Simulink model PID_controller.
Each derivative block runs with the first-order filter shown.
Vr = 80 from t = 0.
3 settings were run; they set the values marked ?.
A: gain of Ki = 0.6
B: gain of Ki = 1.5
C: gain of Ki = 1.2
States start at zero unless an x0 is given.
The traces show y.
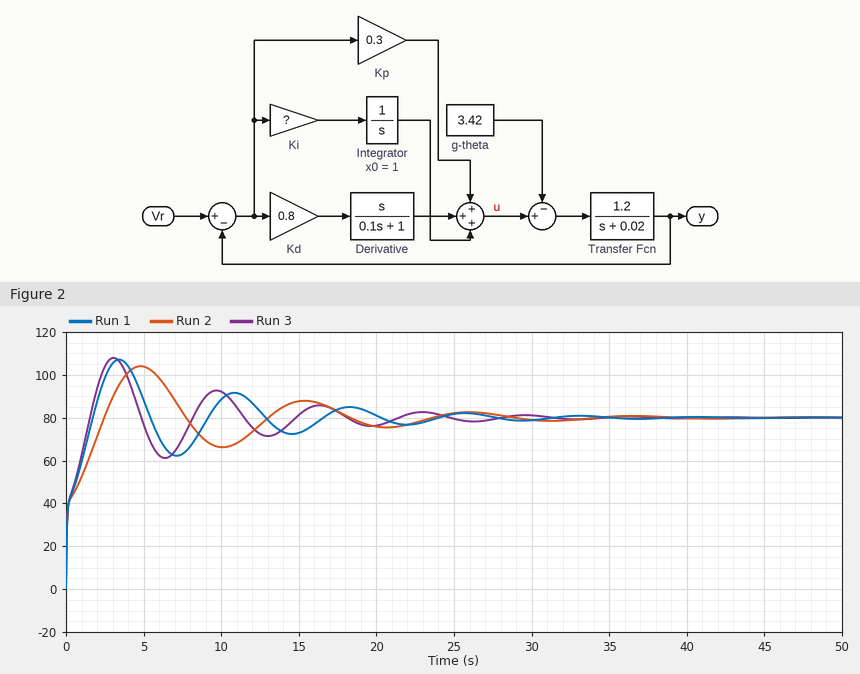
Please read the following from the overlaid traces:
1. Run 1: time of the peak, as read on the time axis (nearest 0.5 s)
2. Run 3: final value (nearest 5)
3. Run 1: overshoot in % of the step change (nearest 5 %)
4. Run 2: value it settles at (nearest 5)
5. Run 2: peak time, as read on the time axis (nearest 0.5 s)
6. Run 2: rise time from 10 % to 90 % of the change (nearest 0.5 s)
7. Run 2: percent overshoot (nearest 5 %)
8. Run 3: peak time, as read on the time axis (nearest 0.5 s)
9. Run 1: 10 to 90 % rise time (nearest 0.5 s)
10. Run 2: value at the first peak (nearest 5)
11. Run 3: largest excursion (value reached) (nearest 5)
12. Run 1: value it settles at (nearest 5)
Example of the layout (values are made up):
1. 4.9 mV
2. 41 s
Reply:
1. 3.5 s
2. 80
3. 35 %
4. 80
5. 5.0 s
6. 2.0 s
7. 30 %
8. 3.0 s
9. 1.5 s
10. 105
11. 110
12. 80
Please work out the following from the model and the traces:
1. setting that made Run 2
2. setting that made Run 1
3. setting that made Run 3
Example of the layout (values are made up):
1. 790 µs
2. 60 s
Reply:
1. A
2. C
3. B
